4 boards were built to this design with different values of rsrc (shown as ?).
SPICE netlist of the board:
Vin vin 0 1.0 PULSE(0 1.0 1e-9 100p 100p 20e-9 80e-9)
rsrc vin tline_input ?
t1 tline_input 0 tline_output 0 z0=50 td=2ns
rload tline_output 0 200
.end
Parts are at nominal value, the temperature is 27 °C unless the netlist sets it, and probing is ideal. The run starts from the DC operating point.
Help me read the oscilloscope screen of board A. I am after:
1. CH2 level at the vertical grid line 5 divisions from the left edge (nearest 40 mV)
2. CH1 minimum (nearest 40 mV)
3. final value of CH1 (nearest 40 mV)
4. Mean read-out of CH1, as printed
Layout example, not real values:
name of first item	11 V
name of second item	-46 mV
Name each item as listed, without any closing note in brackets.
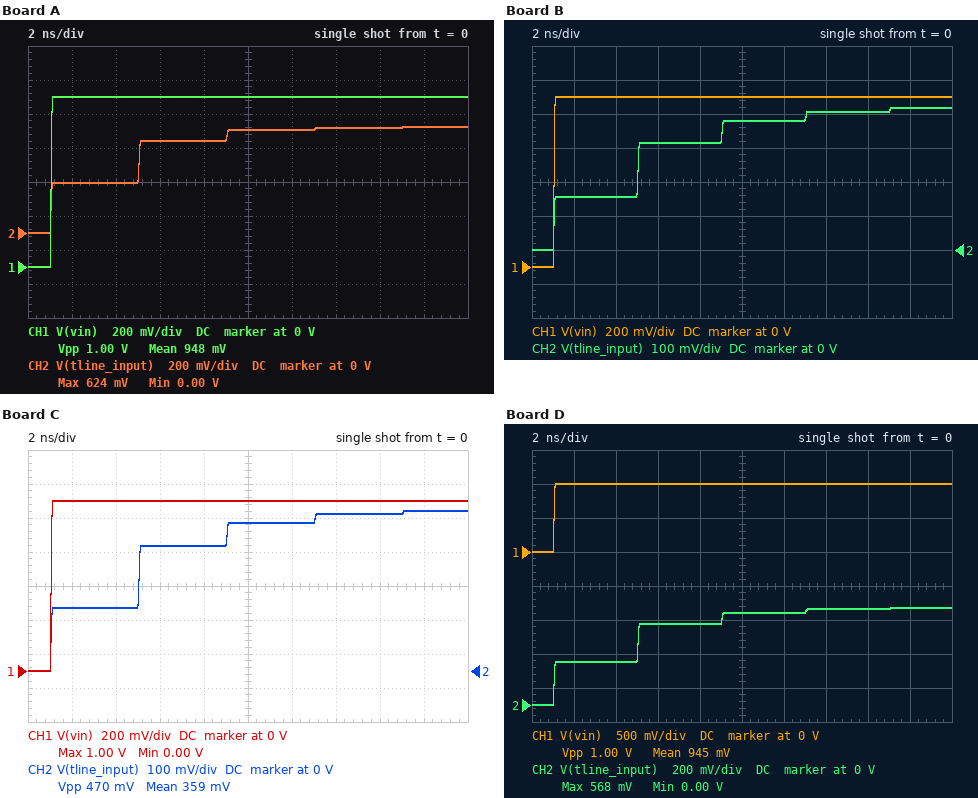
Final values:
CH2 level at the vertical grid line 5 divisions from the left edge	600 mV
CH1 minimum	0 V
final value of CH1	1.00 V
Mean read-out of CH1, as printed	948 mV
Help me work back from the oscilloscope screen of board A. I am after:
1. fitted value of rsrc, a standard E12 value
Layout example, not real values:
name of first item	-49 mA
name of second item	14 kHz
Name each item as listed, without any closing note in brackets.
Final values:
fitted value of rsrc, a standard E12 value	120 Ω
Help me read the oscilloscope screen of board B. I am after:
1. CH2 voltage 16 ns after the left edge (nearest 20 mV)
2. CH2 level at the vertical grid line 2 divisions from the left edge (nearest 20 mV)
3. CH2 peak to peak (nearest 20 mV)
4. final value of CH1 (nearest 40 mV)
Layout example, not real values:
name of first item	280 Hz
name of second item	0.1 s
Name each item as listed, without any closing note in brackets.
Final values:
CH2 voltage 16 ns after the left edge	400 mV
CH2 level at the vertical grid line 2 divisions from the left edge	160 mV
CH2 peak to peak	420 mV
final value of CH1	1.00 V
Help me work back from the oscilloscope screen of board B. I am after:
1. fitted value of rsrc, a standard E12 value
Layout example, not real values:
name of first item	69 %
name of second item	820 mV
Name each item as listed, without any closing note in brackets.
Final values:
fitted value of rsrc, a standard E12 value	270 Ω
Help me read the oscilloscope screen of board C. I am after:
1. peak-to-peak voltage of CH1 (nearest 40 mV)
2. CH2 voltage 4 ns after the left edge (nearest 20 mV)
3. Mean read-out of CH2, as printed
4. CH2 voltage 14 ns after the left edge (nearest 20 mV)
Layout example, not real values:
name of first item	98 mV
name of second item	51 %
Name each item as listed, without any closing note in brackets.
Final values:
peak-to-peak voltage of CH1	1.00 V
CH2 voltage 4 ns after the left edge	180 mV
Mean read-out of CH2, as printed	359 mV
CH2 voltage 14 ns after the left edge	460 mV
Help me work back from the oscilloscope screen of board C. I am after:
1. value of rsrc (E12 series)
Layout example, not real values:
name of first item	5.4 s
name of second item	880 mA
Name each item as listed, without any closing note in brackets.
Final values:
value of rsrc	220 Ω
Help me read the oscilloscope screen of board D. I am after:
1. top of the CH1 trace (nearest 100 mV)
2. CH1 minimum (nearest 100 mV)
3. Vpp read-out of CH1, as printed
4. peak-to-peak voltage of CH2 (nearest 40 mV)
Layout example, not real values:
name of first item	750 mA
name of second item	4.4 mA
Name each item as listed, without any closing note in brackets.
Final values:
top of the CH1 trace	1.0 V
CH1 minimum	0 V
Vpp read-out of CH1, as printed	1.00 V
peak-to-peak voltage of CH2	560 mV
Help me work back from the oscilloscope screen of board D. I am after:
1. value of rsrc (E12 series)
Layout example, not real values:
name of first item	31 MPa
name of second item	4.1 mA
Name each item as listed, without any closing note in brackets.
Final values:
value of rsrc	150 Ω
